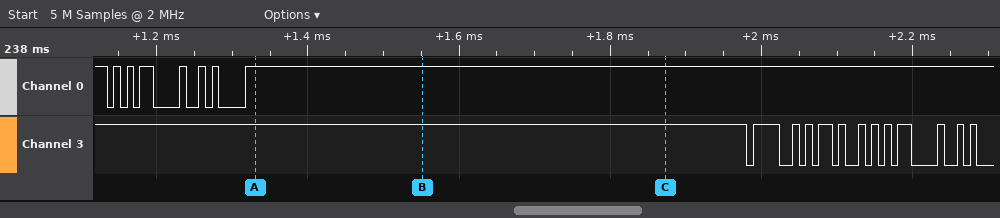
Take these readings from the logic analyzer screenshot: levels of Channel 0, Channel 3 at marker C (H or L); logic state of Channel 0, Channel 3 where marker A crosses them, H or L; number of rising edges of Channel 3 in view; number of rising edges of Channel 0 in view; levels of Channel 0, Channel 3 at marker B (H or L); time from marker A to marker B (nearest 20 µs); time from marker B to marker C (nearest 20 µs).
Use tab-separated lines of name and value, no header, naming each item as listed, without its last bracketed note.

levels of Channel 0, Channel 3 at marker C	Channel 0=H, Channel 3=H
logic state of Channel 0, Channel 3 where marker A crosses them, H or L	Channel 0=H, Channel 3=H
number of rising edges of Channel 3 in view	12
number of rising edges of Channel 0 in view	7
levels of Channel 0, Channel 3 at marker B	Channel 0=H, Channel 3=H
time from marker A to marker B	220 µs
time from marker B to marker C	320 µs
